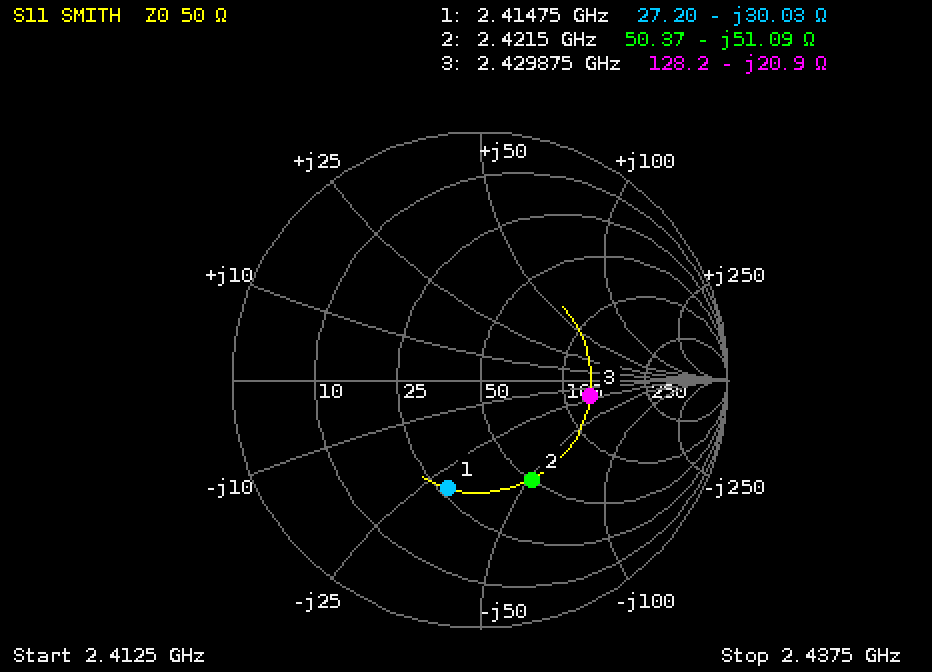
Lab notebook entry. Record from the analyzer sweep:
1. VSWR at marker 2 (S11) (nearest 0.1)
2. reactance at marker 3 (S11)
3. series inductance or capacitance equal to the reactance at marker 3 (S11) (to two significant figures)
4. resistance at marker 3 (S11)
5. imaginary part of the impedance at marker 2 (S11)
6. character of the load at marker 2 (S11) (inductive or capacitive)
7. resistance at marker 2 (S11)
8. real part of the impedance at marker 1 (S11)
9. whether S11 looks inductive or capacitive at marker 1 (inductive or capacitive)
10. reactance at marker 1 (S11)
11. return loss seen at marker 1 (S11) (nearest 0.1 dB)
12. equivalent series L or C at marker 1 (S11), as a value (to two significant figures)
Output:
2.7
-20.9 Ω
3.1 pF
128.2 Ω
-51.09 Ω
capacitive
50.37 Ω
27.20 Ω
capacitive
-30.03 Ω
6.8 dB
2.2 pF
